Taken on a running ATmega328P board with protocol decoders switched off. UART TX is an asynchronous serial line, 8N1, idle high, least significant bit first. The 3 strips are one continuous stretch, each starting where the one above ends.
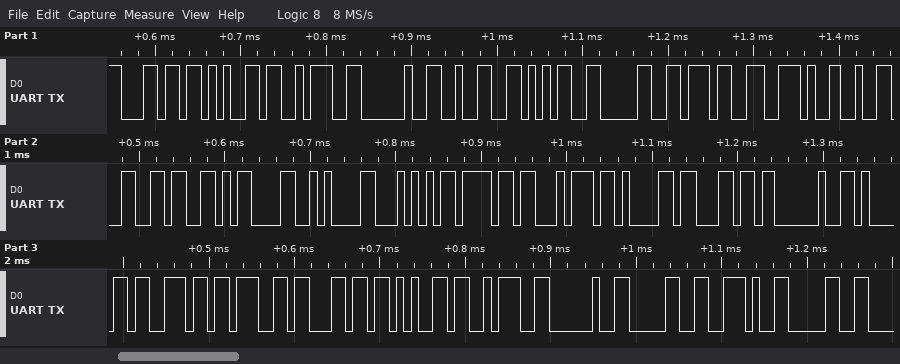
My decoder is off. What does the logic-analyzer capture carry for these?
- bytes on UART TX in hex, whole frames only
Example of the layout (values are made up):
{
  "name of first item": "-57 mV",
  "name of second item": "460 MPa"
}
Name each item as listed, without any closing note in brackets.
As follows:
{
  "bytes on UART TX in hex, whole frames only": "6C 65 3A 20 32 35 30 37 2E 32 36 0D 0A 54 6F 74 61 6C 20 61 6E 67 6C 65 3A 20 30 2E 30"
}
